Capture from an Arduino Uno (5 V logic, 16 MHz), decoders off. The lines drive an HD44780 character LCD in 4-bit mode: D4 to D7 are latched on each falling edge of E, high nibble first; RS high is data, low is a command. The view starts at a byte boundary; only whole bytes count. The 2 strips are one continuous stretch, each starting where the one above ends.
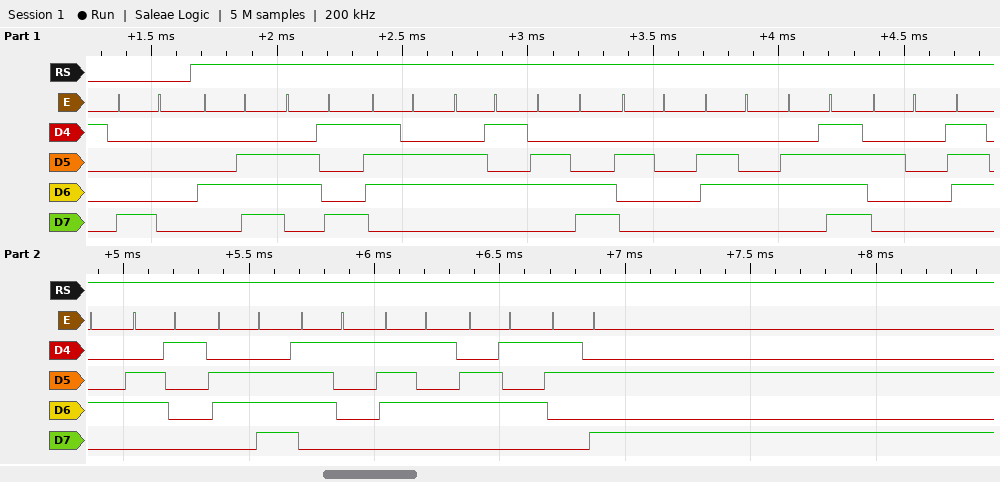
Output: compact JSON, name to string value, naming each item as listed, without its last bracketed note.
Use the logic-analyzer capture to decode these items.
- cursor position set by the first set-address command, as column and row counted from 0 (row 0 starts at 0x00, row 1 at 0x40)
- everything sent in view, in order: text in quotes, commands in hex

{"cursor position set by the first set-address command, as column and row counted from 0": "column 0, row 0", "everything sent in view, in order: text in quotes, commands in hex": "0x80 \"Nivel do tanque:\""}
